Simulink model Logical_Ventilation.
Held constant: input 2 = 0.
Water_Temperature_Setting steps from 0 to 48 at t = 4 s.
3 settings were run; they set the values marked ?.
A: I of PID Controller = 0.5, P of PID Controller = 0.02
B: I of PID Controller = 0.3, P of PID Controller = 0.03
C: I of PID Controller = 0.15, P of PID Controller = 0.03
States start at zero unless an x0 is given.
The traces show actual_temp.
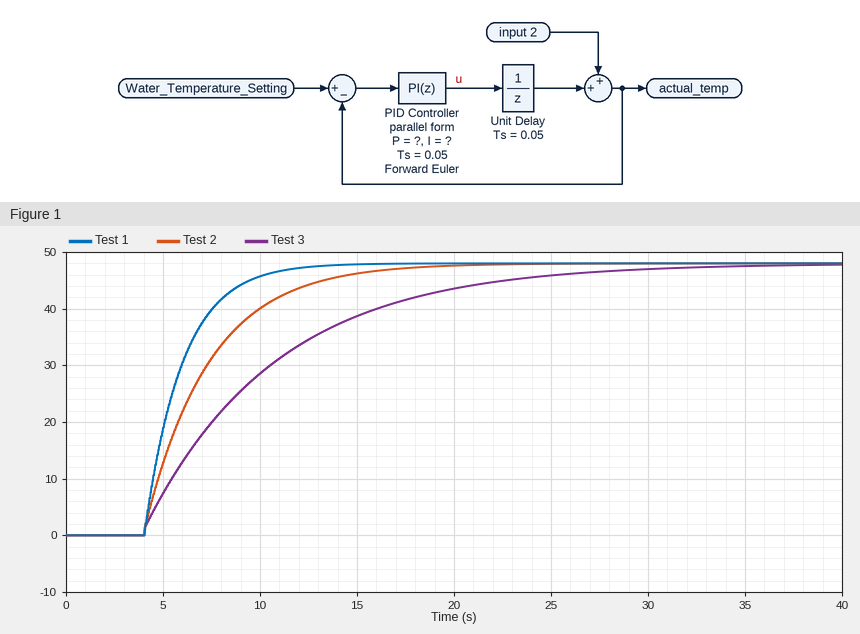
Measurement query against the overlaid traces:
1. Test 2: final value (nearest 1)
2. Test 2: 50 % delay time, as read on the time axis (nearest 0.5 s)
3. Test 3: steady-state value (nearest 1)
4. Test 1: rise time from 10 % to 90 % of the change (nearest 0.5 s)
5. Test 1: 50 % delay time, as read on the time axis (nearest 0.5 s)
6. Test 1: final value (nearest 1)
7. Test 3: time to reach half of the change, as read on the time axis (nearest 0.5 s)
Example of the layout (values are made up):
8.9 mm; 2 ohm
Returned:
48; 6.5 s; 48; 4.5 s; 5.5 s; 48; 8.5 s
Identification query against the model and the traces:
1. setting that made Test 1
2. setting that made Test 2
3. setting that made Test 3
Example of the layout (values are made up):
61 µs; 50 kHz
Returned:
A; B; C
